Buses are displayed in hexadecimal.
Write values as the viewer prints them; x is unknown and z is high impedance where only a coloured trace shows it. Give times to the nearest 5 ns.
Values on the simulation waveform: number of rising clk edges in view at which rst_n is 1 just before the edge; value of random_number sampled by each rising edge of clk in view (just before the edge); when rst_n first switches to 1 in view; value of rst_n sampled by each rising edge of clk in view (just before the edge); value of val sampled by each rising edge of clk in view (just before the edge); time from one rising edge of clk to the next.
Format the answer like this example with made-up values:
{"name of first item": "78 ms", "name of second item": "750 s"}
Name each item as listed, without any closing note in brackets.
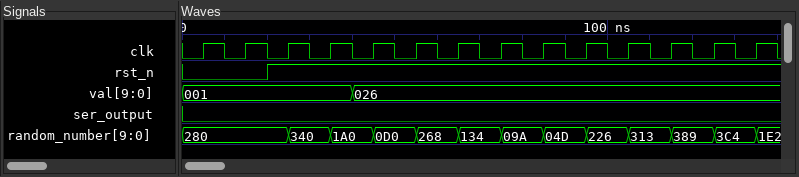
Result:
{"number of rising clk edges in view at which rst_n is 1 just before the edge": "12", "value of random_number sampled by each rising edge of clk in view": "280, 280, 280, 340, 1A0, 0D0, 268, 134, 09A, 04D, 226, 313, 389, 3C4", "when rst_n first switches to 1 in view": "20 ns", "value of rst_n sampled by each rising edge of clk in view": "0 0 1 1 1 1 1 1 1 1 1 1 1 1", "value of val sampled by each rising edge of clk in view": "001, 001, 001, 001, 026, 026, 026, 026, 026, 026, 026, 026, 026, 026", "time from one rising edge of clk to the next": "10 ns"}
